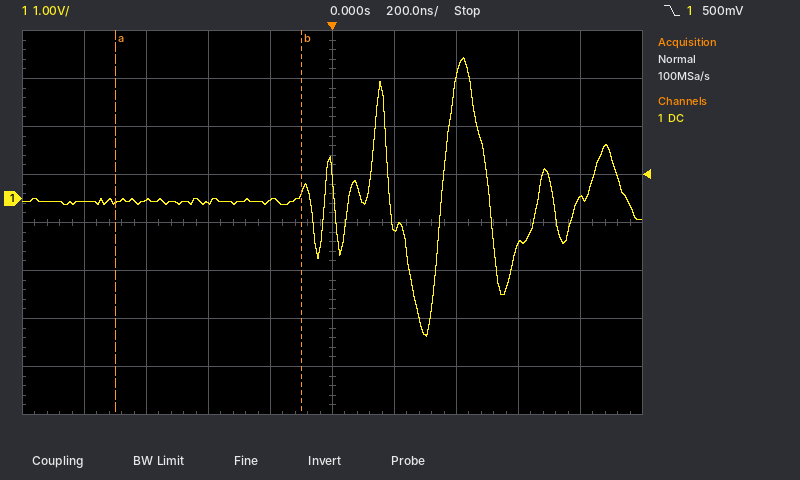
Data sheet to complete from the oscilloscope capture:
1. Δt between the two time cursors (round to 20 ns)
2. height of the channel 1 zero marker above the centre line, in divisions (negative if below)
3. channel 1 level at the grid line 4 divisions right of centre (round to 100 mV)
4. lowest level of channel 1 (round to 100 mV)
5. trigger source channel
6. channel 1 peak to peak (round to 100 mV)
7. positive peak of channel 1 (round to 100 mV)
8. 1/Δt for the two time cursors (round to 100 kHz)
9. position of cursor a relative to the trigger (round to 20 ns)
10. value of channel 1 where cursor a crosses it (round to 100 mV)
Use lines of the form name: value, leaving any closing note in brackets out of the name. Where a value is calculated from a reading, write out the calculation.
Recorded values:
Δt between the two time cursors: 600 ns
height of the channel 1 zero marker above the centre line, in divisions: +0.5 div
channel 1 level at the grid line 4 divisions right of centre: 0.0 V
lowest level of channel 1: -2.9 V
trigger source channel: channel 1
channel 1 peak to peak: 2.9 V − (-2.9 V) = 5.8 V
positive peak of channel 1: 2.9 V
1/Δt for the two time cursors: 1 / 600 ns ≈ 1.7 MHz
position of cursor a relative to the trigger: -700 ns
value of channel 1 where cursor a crosses it: -100 mV
